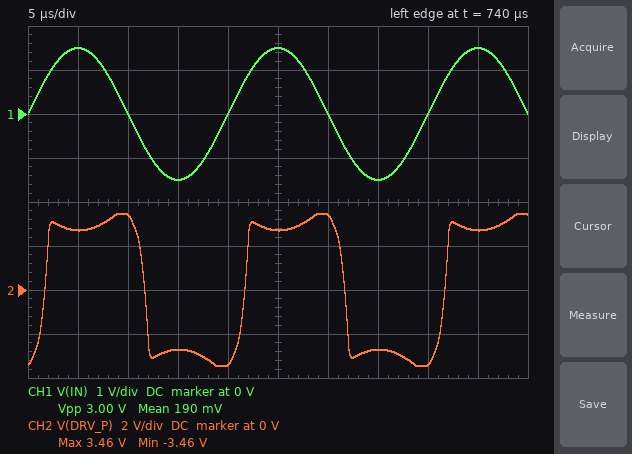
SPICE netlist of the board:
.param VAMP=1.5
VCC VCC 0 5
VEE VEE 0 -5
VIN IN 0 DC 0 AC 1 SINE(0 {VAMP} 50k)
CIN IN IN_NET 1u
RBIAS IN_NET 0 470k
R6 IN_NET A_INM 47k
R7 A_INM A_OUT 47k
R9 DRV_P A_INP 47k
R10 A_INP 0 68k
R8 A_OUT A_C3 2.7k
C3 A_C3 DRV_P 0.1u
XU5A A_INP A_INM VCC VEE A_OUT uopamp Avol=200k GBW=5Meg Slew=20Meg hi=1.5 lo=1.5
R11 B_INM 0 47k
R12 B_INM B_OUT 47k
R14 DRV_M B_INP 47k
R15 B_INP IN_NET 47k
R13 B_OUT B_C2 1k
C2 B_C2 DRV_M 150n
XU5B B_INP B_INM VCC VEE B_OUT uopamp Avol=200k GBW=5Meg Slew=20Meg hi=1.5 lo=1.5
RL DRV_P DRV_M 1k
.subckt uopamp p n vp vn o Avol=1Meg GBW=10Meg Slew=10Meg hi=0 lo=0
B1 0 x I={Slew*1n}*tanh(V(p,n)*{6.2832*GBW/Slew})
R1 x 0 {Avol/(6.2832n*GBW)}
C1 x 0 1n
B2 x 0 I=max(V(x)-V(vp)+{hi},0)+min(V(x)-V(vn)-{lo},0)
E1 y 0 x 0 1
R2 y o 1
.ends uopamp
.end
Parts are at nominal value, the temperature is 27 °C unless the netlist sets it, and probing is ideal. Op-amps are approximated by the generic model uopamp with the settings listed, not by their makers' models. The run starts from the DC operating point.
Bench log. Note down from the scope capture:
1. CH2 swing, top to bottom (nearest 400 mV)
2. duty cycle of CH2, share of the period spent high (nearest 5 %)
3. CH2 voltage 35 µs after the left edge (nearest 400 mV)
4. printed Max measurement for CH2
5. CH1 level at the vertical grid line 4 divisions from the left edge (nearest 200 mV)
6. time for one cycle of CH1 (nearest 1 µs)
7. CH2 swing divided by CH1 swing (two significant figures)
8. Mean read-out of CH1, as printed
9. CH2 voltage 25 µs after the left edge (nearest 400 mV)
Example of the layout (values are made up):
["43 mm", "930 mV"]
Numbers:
["6.8 V", "50 %", "-2.8 V", "3.46 V", "0 V", "20 µs", "2.3", "190 mV", "2.8 V"]
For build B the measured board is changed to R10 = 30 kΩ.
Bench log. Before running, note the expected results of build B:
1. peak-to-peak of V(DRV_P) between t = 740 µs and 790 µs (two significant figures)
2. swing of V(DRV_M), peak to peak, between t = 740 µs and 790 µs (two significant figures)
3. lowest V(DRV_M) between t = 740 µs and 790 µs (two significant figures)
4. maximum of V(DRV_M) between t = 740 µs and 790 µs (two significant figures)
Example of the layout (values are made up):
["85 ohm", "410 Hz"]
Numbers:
["5.2 V", "6.1 V", "-3.0 V", "3.0 V"]
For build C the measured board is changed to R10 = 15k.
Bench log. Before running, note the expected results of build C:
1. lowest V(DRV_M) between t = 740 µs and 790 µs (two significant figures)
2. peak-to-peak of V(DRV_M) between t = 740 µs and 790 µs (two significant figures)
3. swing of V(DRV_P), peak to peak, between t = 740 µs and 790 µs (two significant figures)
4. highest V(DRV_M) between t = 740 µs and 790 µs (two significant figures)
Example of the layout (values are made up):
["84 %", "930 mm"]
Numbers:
["-2.8 V", "5.5 V", "4.1 V", "2.8 V"]
